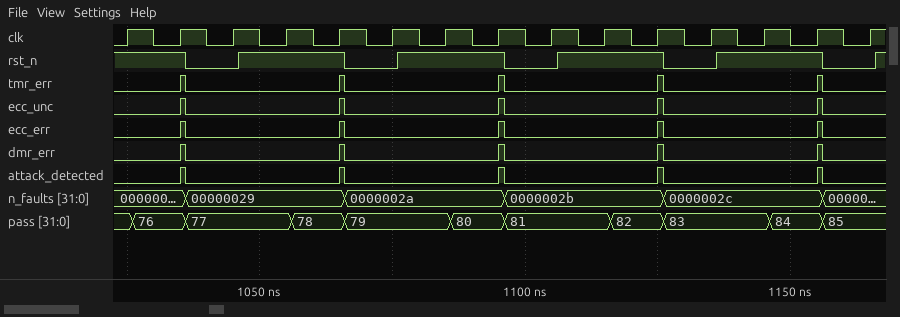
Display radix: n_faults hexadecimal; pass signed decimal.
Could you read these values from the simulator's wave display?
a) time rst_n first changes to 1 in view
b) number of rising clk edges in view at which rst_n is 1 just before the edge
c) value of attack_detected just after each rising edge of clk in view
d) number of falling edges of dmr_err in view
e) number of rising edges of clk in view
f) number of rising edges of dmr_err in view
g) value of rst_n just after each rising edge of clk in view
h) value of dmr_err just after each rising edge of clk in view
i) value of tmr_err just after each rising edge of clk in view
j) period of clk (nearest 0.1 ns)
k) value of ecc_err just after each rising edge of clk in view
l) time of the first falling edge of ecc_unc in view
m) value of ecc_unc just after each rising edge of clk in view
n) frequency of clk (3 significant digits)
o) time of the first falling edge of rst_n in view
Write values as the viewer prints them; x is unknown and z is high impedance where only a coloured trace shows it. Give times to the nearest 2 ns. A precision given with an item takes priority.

1046 ns
10
0 1 0 0 1 0 0 1 0 0 1 0 0 1 0
5
15
5
1 1 0 1 1 0 1 1 0 1 1 0 1 1 0
0 1 0 0 1 0 0 1 0 0 1 0 0 1 0
0 1 0 0 1 0 0 1 0 0 1 0 0 1 0
10 ns
0 1 0 0 1 0 0 1 0 0 1 0 0 1 0
1036 ns
0 1 0 0 1 0 0 1 0 0 1 0 0 1 0
100 MHz
1036 ns
